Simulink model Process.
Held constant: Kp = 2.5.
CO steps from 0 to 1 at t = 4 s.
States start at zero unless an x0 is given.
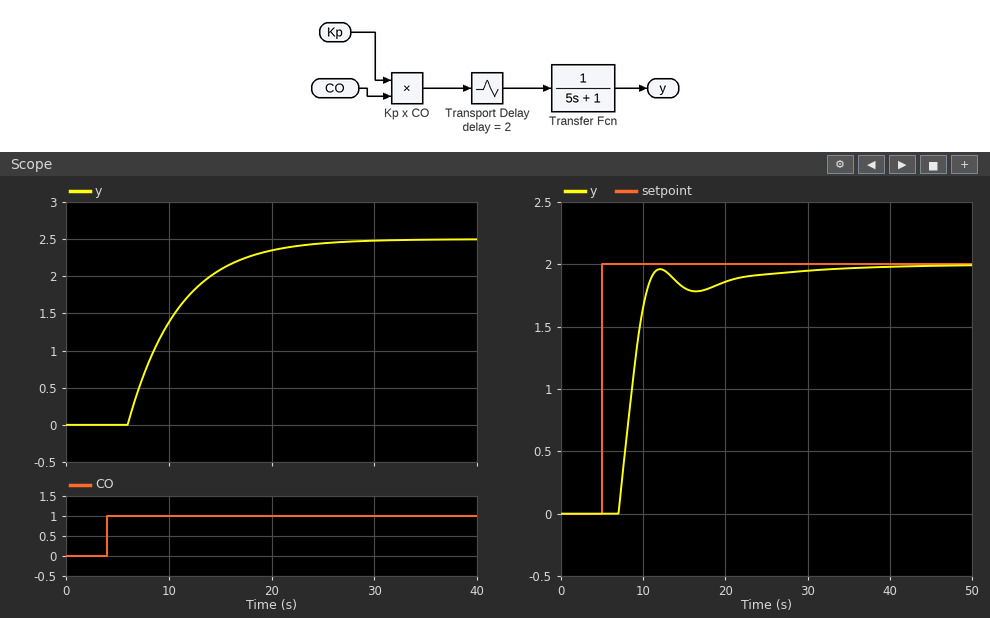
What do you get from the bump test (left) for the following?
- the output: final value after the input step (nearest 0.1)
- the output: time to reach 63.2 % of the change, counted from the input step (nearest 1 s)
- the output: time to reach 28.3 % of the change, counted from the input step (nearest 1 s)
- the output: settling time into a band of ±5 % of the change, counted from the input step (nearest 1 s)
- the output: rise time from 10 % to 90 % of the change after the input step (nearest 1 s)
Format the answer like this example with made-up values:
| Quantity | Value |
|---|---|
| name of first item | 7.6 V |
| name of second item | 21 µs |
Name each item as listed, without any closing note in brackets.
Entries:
| Quantity | Value |
|---|---|
| the output: final value after the input step | 2.5 |
| the output: time to reach 63.2 % of the change, counted from the input step | 7 s |
| the output: time to reach 28.3 % of the change, counted from the input step | 4 s |
| the output: settling time into a band of ±5 % of the change, counted from the input step | 17 s |
| the output: rise time from 10 % to 90 % of the change after the input step | 11 s |
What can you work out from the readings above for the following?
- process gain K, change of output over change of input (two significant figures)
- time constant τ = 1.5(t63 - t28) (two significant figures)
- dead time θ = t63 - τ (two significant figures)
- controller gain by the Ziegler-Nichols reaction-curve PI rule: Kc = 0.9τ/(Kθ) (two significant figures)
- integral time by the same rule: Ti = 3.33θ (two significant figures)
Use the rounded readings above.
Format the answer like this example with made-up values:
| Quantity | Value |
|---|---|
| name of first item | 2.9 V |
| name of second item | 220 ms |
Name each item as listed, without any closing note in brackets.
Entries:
| Quantity | Value |
|---|---|
| process gain K, change of output over change of input | 2.5 |
| time constant τ = 1.5(t63 - t28) | 4.5 s |
| dead time θ = t63 - τ | 2.5 s |
| controller gain by the Ziegler-Nichols reaction-curve PI rule: Kc = 0.9τ/(Kθ) | 0.65 |
| integral time by the same rule: Ti = 3.33θ | 8.3 s |
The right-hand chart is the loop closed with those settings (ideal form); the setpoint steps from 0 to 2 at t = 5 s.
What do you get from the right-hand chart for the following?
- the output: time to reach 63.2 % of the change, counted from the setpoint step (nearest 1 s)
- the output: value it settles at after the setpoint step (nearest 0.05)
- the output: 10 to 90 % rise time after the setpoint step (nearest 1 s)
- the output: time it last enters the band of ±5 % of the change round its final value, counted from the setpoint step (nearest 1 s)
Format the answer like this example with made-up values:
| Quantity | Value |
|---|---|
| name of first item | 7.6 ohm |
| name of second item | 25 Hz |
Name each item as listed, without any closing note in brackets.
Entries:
| Quantity | Value |
|---|---|
| the output: time to reach 63.2 % of the change, counted from the setpoint step | 4 s |
| the output: value it settles at after the setpoint step | 2.00 |
| the output: 10 to 90 % rise time after the setpoint step | 3 s |
| the output: time it last enters the band of ±5 % of the change round its final value, counted from the setpoint step | 17 s |
